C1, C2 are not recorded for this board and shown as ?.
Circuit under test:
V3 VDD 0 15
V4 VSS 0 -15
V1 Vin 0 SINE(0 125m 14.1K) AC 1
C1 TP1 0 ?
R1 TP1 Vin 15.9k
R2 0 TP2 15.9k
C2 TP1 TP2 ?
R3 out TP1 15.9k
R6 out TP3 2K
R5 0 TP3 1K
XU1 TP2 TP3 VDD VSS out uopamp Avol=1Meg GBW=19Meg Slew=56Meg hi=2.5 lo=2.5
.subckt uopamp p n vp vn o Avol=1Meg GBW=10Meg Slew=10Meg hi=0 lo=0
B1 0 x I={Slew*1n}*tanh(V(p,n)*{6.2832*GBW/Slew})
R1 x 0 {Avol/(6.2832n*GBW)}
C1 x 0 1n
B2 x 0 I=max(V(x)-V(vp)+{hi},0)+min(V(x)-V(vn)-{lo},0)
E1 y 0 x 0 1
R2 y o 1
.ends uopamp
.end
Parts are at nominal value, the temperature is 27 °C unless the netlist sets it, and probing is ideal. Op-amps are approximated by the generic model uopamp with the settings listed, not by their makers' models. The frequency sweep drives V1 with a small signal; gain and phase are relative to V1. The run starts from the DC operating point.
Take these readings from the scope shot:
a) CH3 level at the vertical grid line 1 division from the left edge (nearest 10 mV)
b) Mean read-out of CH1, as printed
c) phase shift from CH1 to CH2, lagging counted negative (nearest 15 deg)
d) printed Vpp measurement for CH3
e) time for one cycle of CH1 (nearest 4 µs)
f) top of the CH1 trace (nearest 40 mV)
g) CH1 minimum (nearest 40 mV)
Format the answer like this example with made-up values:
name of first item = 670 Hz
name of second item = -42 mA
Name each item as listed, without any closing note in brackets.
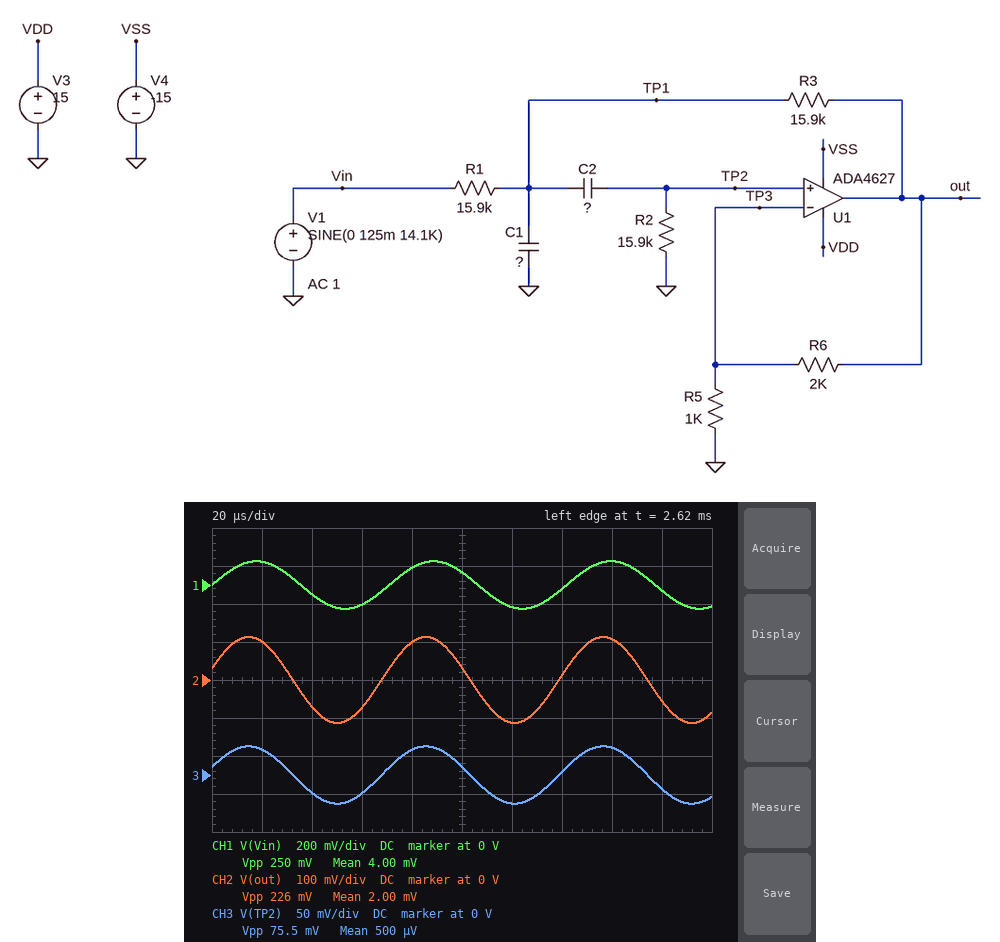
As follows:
CH3 level at the vertical grid line 1 division from the left edge = 30 mV
Mean read-out of CH1, as printed = 4.00 mV
phase shift from CH1 to CH2, lagging counted negative = 15 deg
printed Vpp measurement for CH3 = 75.5 mV
time for one cycle of CH1 = 72 µs
top of the CH1 trace = 120 mV
CH1 minimum = -120 mV
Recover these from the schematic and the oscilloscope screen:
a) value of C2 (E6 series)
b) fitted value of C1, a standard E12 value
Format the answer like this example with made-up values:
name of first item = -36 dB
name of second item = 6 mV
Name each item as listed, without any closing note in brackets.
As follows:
value of C2 = 470 pF
fitted value of C1, a standard E12 value = 1.5 nF
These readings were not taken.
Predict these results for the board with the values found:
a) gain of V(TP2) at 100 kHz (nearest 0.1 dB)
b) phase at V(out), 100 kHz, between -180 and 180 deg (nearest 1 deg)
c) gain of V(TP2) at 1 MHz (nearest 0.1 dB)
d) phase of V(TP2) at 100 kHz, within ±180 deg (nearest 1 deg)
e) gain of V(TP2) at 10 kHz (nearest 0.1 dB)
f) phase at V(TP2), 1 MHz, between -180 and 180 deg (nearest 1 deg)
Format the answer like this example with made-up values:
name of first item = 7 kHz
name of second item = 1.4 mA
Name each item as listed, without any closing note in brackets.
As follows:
gain of V(TP2) at 100 kHz = -23.5 dB
phase at V(out), 100 kHz, between -180 and 180 deg = -79 deg
gain of V(TP2) at 1 MHz = -43.5 dB
phase of V(TP2) at 100 kHz, within ±180 deg = -78 deg
gain of V(TP2) at 10 kHz = -12.5 dB
phase at V(TP2), 1 MHz, between -180 and 180 deg = -89 deg
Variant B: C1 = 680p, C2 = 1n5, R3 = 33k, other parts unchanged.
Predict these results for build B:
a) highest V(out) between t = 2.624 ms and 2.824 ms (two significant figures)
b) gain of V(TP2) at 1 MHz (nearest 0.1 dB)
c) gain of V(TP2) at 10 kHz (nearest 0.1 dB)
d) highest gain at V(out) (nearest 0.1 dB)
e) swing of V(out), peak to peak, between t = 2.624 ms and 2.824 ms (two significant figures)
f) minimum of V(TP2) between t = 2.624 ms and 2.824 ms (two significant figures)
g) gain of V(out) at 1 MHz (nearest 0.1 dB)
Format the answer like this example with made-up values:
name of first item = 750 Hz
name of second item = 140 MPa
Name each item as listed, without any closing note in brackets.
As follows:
highest V(out) between t = 2.624 ms and 2.824 ms = 250 mV
gain of V(TP2) at 1 MHz = -36.7 dB
gain of V(TP2) at 10 kHz = -3.6 dB
highest gain at V(out) = 6.1 dB
swing of V(out), peak to peak, between t = 2.624 ms and 2.824 ms = 500 mV
minimum of V(TP2) between t = 2.624 ms and 2.824 ms = -83 mV
gain of V(out) at 1 MHz = -27.2 dB
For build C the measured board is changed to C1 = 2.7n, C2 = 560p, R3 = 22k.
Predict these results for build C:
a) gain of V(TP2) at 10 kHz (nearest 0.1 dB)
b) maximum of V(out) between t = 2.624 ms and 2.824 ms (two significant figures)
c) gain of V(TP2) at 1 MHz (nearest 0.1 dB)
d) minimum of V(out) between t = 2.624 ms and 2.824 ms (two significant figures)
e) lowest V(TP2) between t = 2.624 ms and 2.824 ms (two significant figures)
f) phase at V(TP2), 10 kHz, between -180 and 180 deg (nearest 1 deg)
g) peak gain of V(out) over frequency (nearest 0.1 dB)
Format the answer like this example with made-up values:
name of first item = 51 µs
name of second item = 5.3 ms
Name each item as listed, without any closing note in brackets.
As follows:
gain of V(TP2) at 10 kHz = -14.6 dB
maximum of V(out) between t = 2.624 ms and 2.824 ms = 67 mV
gain of V(TP2) at 1 MHz = -48.6 dB
minimum of V(out) between t = 2.624 ms and 2.824 ms = -67 mV
lowest V(TP2) between t = 2.624 ms and 2.824 ms = -22 mV
phase at V(TP2), 10 kHz, between -180 and 180 deg = 4 deg
peak gain of V(out) over frequency = -5.1 dB
